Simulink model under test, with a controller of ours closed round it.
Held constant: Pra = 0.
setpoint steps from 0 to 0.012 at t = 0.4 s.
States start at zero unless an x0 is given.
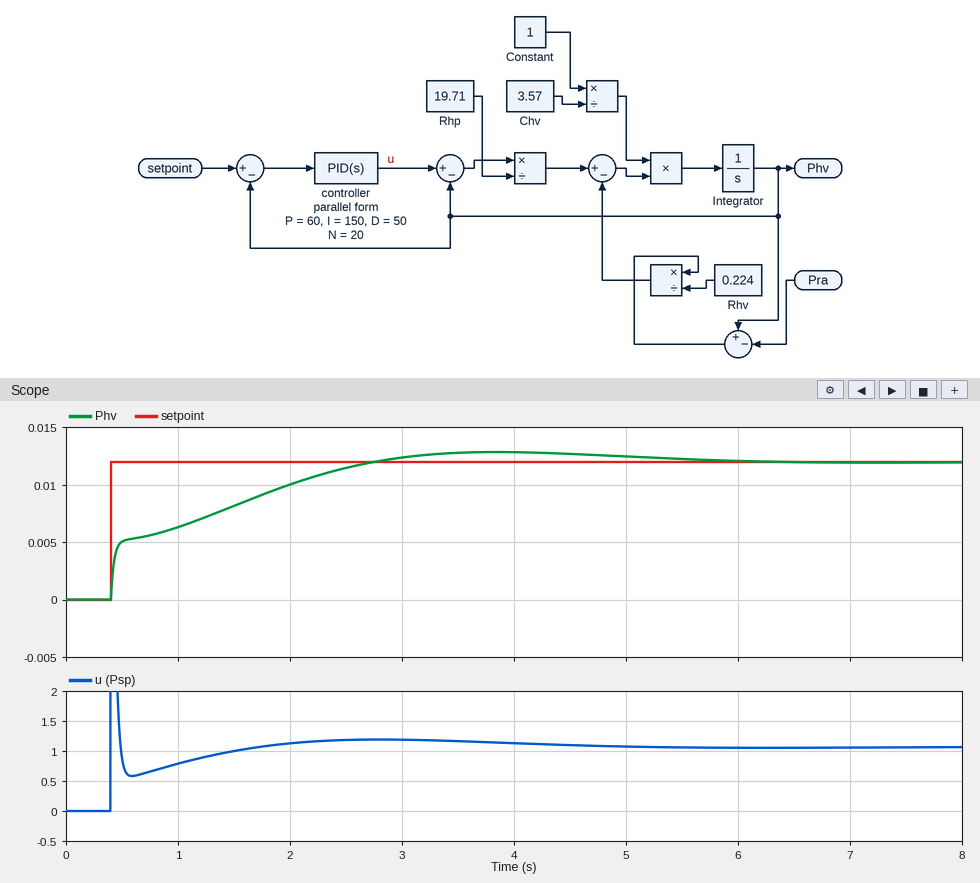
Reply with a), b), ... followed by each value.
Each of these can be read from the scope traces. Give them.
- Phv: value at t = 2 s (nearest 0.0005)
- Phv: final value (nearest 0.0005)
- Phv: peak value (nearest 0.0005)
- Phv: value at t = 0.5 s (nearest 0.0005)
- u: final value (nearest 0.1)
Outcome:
a) 0.0100
b) 0.0120
c) 0.0130
d) 0.0050
e) 1.1
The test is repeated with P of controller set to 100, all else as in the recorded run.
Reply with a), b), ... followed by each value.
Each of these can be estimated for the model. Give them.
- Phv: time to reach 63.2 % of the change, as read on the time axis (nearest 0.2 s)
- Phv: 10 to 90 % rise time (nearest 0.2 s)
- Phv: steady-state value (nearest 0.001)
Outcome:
a) 1.2 s
b) 1.8 s
c) 0.012
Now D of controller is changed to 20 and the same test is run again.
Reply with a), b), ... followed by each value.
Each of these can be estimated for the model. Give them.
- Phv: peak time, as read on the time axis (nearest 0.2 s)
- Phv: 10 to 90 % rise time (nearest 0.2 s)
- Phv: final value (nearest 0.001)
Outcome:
a) 3.4 s
b) 1.6 s
c) 0.012
